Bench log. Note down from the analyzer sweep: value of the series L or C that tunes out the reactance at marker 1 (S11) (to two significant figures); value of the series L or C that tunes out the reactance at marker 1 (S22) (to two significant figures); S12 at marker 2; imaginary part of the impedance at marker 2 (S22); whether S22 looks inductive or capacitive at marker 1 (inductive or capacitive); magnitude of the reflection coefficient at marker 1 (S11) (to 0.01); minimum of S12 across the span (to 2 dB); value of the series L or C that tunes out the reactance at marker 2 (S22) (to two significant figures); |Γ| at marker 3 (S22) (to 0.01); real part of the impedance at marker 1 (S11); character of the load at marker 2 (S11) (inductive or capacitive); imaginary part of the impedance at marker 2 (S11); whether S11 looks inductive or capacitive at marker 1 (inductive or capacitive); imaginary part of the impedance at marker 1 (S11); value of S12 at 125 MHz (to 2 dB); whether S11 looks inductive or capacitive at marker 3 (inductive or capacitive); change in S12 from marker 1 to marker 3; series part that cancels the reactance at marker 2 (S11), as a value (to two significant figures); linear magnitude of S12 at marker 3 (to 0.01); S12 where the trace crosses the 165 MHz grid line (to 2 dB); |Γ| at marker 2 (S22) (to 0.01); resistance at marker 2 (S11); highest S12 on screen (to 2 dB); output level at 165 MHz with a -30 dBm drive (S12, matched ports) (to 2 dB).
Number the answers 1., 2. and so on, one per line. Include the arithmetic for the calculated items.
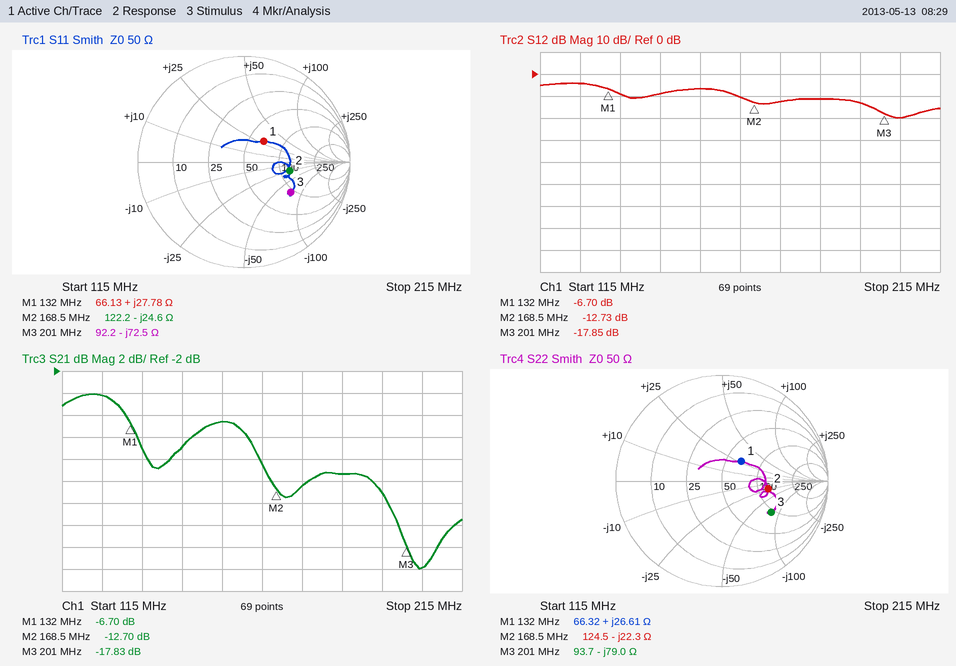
1. C = 1/(2π × 132 MHz × 27.78 Ω) ≈ 43 pF
2. C = 1/(2π × 132 MHz × 26.61 Ω) ≈ 45 pF
3. -12.73 dB
4. -22.3 Ω
5. inductive
6. 0.27
7. -20 dB
8. L = 22.3 Ω/(2π × 168.5 MHz) ≈ 21 nH
9. 0.55
10. 66.13 Ω
11. capacitive
12. -24.6 Ω
13. inductive
14. +27.78 Ω
15. -4 dB
16. capacitive
17. -17.85 − (-6.7) = -11.15 dB
18. L = 24.6 Ω/(2π × 168.5 MHz) ≈ 23 nH
19. 10^(-17.85/20) ≈ 0.13
20. -10 dB
21. 0.44
22. 122.2 Ω
23. -4 dB
24. -30 dBm + (-10 dB) = -40 dBm
